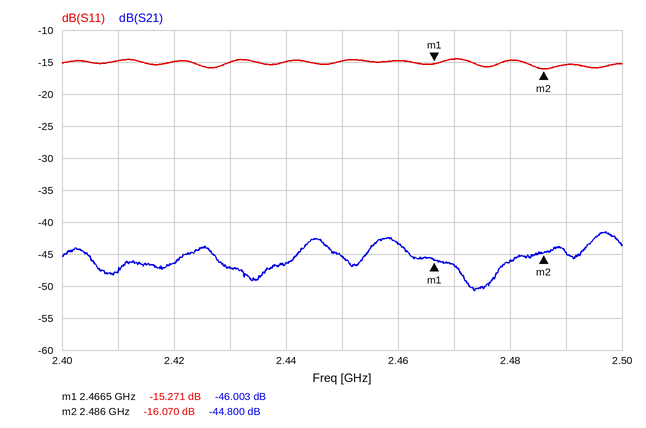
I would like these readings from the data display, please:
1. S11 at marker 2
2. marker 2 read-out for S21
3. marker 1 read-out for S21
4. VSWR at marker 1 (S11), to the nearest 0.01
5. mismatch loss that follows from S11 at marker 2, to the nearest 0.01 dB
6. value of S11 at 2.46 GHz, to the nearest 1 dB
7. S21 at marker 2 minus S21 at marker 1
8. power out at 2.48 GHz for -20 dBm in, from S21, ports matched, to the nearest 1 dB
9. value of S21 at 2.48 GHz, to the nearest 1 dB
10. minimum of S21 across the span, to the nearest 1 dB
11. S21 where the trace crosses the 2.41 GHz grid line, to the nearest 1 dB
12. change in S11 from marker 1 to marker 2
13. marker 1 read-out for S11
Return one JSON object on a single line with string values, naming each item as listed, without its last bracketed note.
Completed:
{"S11 at marker 2": "-16.070 dB", "marker 2 read-out for S21": "-44.800 dB", "marker 1 read-out for S21": "-46.003 dB", "VSWR at marker 1 (S11), to the nearest 0.01": "1.42", "mismatch loss that follows from S11 at marker 2, to the nearest 0.01 dB": "0.11 dB", "value of S11 at 2.46 GHz, to the nearest 1 dB": "-15 dB", "S21 at marker 2 minus S21 at marker 1": "1.203 dB", "power out at 2.48 GHz for -20 dBm in, from S21, ports matched, to the nearest 1 dB": "-66 dBm", "value of S21 at 2.48 GHz, to the nearest 1 dB": "-46 dB", "minimum of S21 across the span, to the nearest 1 dB": "-51 dB", "S21 where the trace crosses the 2.41 GHz grid line, to the nearest 1 dB": "-48 dB", "change in S11 from marker 1 to marker 2": "-0.799 dB", "marker 1 read-out for S11": "-15.271 dB"}
